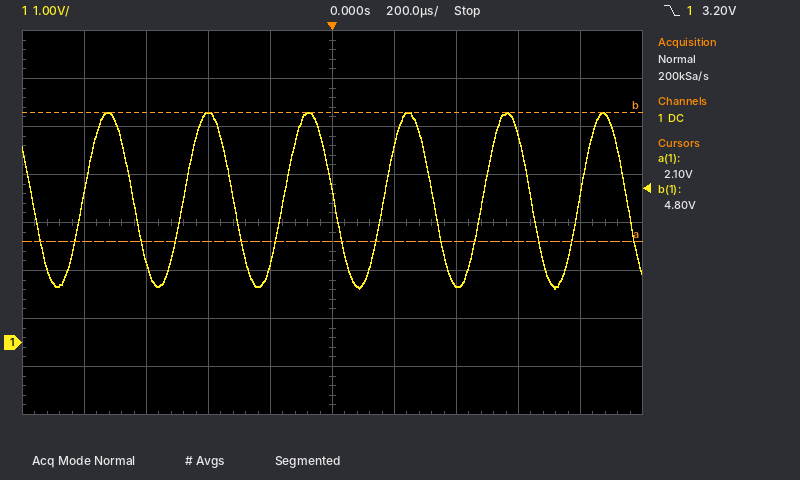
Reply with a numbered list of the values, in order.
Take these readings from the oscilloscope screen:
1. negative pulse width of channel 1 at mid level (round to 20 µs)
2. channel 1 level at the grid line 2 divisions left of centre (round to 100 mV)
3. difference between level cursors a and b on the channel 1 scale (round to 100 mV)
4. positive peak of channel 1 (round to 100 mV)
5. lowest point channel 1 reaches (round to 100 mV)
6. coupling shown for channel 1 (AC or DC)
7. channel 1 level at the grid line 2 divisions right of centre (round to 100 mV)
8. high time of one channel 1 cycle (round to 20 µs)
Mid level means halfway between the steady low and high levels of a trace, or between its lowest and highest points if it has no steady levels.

1. 160 µs
2. 4.8 V
3. 2.7 V
4. 4.8 V
5. 1.1 V
6. DC
7. 1.2 V
8. 160 µs
